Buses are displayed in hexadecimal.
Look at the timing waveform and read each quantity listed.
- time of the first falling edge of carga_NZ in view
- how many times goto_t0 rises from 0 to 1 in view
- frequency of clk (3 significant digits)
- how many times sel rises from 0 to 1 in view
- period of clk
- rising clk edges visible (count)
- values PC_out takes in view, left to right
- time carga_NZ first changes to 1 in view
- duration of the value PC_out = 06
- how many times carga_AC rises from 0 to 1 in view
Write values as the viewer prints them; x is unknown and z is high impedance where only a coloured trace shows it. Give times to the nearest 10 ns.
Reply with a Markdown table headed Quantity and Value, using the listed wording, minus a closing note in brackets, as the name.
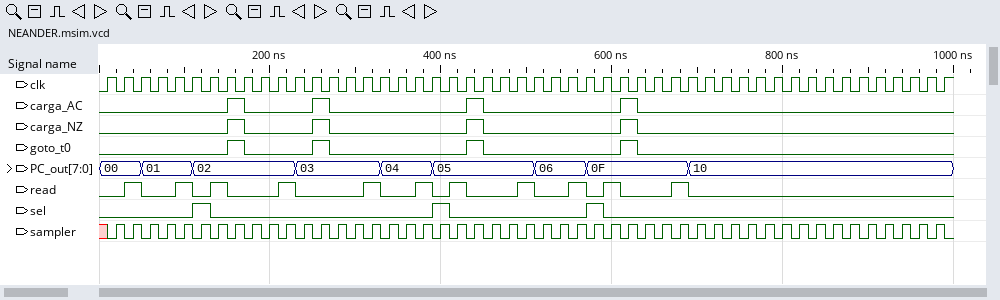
| Quantity | Value |
|---|---|
| time of the first falling edge of carga_NZ in view | 170 ns |
| how many times goto_t0 rises from 0 to 1 in view | 4 |
| frequency of clk | 50.0 MHz |
| how many times sel rises from 0 to 1 in view | 3 |
| period of clk | 20 ns |
| rising clk edges visible | 50 |
| values PC_out takes in view, left to right | 00, 01, 02, 03, 04, 05, 06, 0F, 10 |
| time carga_NZ first changes to 1 in view | 150 ns |
| duration of the value PC_out = 06 | 60 ns |
| how many times carga_AC rises from 0 to 1 in view | 4 |
